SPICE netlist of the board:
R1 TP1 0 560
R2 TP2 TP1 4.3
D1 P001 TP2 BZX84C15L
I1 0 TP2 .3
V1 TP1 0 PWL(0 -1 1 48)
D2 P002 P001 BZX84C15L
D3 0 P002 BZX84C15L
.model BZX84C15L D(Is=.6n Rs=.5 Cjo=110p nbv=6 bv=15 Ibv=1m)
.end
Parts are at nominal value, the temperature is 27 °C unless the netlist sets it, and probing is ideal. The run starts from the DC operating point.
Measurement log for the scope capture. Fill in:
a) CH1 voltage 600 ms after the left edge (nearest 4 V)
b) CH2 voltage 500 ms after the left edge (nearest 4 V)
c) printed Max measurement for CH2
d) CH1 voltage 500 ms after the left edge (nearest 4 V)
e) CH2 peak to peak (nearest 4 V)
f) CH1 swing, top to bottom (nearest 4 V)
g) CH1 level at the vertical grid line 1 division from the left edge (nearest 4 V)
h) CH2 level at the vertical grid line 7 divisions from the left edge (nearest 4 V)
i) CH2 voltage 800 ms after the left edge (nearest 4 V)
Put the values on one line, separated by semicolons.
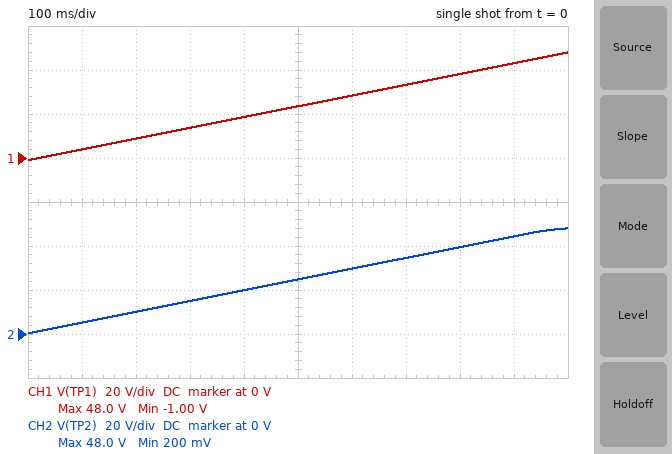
28 V; 24 V; 48.0 V; 24 V; 48 V; 48 V; 4 V; 36 V; 40 V
